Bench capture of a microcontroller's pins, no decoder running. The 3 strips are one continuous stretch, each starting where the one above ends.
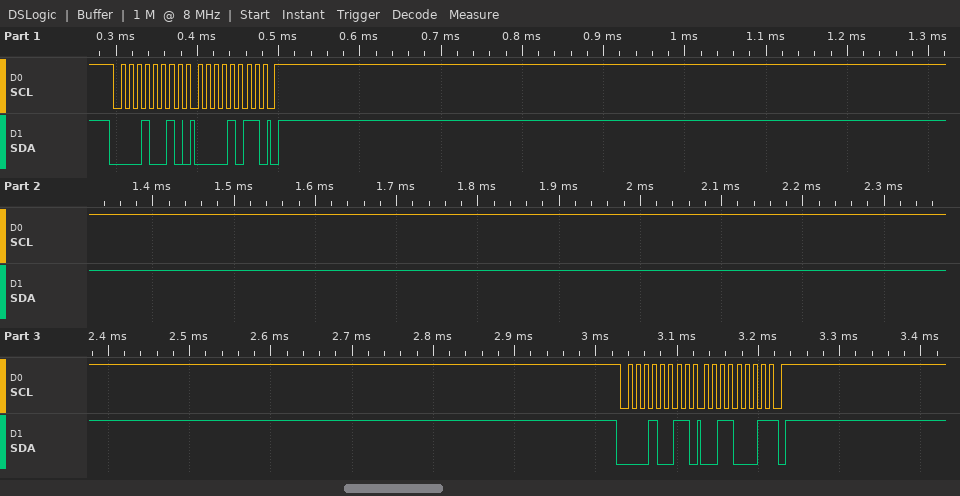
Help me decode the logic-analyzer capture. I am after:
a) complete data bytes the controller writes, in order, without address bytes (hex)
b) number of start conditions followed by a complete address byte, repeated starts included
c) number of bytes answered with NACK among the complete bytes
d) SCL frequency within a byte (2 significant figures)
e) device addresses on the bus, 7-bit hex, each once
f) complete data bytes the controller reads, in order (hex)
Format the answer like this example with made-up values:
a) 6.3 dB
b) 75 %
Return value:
a) 0B
b) 2
c) 1
d) 100 kHz
e) 0x09
f) 31
